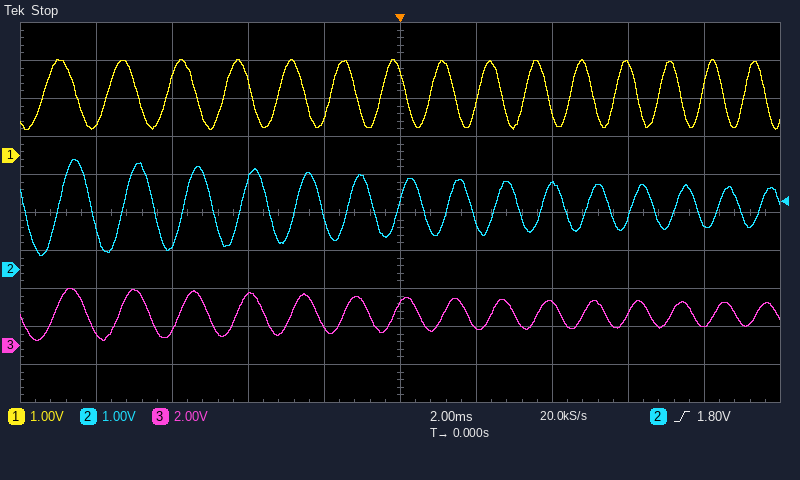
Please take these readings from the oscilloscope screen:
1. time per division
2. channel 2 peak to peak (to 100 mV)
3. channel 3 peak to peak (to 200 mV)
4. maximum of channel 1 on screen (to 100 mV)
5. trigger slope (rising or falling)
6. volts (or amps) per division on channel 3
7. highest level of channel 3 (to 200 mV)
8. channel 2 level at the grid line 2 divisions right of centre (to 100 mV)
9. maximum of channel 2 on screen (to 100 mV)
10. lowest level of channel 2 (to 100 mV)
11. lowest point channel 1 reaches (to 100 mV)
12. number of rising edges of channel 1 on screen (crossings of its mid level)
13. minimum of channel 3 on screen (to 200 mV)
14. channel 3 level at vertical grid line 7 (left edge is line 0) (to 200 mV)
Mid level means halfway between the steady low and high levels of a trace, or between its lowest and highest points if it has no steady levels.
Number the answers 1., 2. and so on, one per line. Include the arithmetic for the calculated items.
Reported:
1. 2 ms
2. 2.9 V − (400 mV) = 2.5 V
3. 3.0 V − (200 mV) = 2.8 V
4. 2.5 V
5. rising
6. 2 V
7. 3.0 V
8. 2.2 V
9. 2.9 V
10. 400 mV
11. 700 mV
12. 15
13. 200 mV
14. 2.2 V
